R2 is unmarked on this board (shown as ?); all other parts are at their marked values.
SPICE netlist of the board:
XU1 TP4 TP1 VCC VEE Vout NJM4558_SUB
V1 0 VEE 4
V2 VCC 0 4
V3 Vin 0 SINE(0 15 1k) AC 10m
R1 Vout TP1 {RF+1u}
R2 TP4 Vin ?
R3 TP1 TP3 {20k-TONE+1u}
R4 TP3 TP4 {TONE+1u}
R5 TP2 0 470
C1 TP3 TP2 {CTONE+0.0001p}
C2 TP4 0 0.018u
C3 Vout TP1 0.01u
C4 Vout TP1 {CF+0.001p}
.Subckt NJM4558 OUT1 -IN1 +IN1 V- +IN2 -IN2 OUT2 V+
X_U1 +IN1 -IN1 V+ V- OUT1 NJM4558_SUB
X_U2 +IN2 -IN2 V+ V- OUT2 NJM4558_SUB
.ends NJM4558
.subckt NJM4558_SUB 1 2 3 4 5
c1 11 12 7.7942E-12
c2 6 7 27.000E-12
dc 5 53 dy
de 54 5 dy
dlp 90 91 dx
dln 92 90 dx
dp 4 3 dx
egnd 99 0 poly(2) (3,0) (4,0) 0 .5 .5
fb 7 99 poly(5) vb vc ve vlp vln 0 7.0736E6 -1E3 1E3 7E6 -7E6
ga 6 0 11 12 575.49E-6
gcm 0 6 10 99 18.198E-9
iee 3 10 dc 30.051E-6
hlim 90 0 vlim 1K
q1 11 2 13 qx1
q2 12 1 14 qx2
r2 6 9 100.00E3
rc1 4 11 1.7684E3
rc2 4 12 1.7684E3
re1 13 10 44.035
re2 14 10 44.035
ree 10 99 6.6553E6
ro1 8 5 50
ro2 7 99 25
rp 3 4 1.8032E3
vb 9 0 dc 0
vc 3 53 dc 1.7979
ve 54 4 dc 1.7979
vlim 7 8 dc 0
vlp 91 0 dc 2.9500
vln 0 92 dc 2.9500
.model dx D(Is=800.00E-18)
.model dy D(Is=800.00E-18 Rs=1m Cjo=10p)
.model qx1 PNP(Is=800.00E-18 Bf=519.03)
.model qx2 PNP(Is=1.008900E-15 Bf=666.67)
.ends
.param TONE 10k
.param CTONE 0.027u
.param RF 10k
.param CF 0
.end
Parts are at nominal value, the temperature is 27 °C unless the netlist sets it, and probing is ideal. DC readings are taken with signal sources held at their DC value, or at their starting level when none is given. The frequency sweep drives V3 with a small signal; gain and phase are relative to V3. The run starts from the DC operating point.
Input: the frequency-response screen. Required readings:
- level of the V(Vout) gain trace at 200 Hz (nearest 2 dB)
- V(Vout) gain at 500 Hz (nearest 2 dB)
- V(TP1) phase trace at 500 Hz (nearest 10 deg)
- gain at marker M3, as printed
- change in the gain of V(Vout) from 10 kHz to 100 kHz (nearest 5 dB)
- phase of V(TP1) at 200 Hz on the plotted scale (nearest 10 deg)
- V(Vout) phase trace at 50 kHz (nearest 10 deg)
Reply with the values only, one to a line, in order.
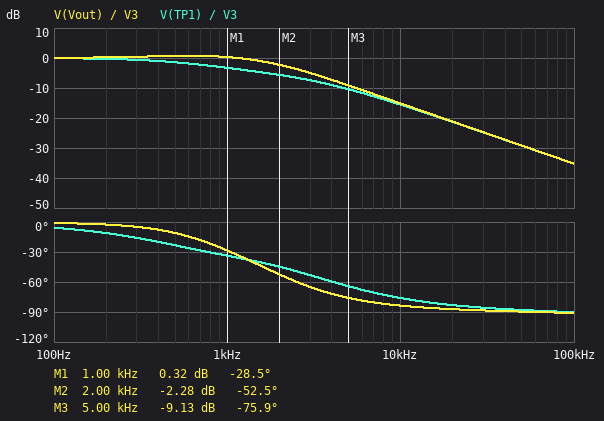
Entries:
0 dB
0 dB
-20 deg
-9.13 dB
-20 dB
-10 deg
-90 deg
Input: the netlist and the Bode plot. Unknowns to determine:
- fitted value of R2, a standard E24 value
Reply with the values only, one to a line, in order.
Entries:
5.1 kΩ
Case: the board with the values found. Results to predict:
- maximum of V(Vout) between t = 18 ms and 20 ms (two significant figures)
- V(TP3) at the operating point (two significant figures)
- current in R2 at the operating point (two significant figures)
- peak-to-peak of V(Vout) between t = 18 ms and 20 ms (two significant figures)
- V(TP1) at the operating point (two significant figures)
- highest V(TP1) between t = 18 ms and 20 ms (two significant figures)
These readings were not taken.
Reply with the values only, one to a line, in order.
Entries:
3.0 V
-4.4 mV
280 nA
5.9 V
-7.4 mV
5.2 V
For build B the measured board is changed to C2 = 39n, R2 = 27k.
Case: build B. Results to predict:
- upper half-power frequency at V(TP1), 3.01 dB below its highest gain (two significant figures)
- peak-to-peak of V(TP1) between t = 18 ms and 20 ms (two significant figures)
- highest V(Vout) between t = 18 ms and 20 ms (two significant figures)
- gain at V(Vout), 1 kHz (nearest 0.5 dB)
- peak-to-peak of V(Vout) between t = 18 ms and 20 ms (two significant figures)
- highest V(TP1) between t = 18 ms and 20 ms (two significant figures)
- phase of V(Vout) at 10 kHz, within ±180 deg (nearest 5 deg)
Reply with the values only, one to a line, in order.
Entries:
110 Hz
3.7 V
2.8 V
-14.5 dB
5.6 V
1.8 V
-95 deg
